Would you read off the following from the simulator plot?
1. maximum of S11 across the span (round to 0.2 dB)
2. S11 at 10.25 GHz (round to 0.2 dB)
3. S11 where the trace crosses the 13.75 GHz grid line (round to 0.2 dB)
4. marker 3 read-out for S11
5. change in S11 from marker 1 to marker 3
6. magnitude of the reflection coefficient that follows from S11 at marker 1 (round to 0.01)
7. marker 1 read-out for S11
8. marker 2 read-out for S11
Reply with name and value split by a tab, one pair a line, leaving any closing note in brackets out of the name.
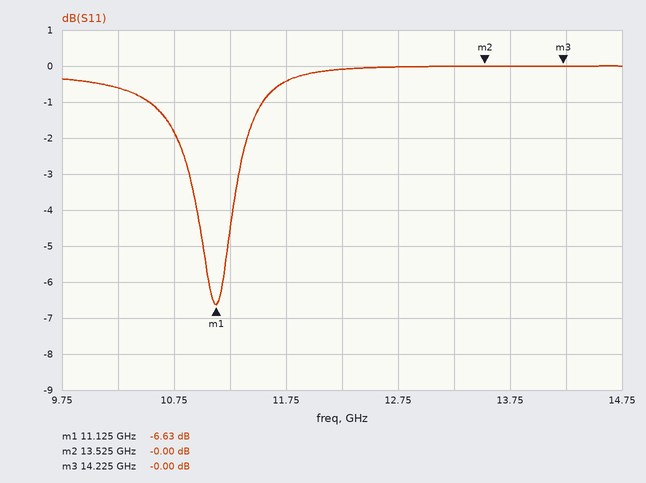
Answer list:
maximum of S11 across the span	0.0 dB
S11 at 10.25 GHz	-0.6 dB
S11 where the trace crosses the 13.75 GHz grid line	0.0 dB
marker 3 read-out for S11	-0.00 dB
change in S11 from marker 1 to marker 3	6.63 dB
magnitude of the reflection coefficient that follows from S11 at marker 1	0.47
marker 1 read-out for S11	-6.63 dB
marker 2 read-out for S11	-0.00 dB
